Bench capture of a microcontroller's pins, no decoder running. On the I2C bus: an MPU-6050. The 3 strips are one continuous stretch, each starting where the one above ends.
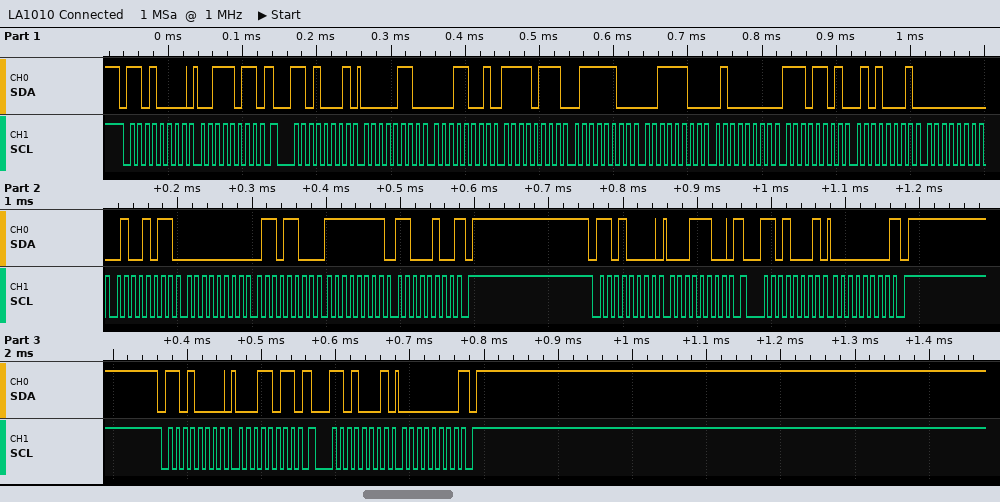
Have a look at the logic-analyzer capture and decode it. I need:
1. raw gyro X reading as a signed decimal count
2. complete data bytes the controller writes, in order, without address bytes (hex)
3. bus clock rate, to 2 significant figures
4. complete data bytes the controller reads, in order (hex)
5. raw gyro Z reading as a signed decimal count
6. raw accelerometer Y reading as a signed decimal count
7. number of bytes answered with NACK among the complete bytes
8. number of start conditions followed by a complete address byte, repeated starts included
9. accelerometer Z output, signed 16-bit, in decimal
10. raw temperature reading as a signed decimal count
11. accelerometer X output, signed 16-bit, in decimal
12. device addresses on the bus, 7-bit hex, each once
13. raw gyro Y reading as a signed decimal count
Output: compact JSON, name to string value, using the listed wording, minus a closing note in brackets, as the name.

{"raw gyro X reading as a signed decimal count": "75", "complete data bytes the controller writes, in order, without address bytes": "3B 1C 1B", "bus clock rate, to 2 significant figures": "100 kHz", "complete data bytes the controller reads, in order": "06 19 F7 7C 3C 40 ED 51 00 4B 00 6C FF C4 00 00", "raw gyro Z reading as a signed decimal count": "-60", "raw accelerometer Y reading as a signed decimal count": "-2180", "number of bytes answered with NACK among the complete bytes": "3", "number of start conditions followed by a complete address byte, repeated starts included": "6", "accelerometer Z output, signed 16-bit, in decimal": "15424", "raw temperature reading as a signed decimal count": "-4783", "accelerometer X output, signed 16-bit, in decimal": "1561", "device addresses on the bus, 7-bit hex, each once": "0x68", "raw gyro Y reading as a signed decimal count": "108"}
